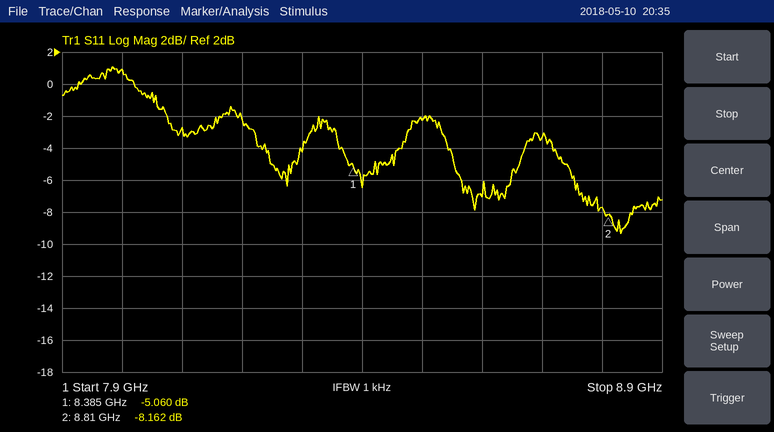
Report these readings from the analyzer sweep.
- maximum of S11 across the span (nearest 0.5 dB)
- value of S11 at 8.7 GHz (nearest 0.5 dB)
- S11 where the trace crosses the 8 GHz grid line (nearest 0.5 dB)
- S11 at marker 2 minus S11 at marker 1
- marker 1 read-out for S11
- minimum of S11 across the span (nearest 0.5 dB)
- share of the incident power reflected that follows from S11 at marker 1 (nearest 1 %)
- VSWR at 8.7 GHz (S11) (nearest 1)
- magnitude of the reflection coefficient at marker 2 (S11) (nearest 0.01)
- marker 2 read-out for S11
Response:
1.0 dB
-3.5 dB
1.0 dB
-3.102 dB
-5.060 dB
-9.5 dB
31 %
5
0.39
-8.162 dB
